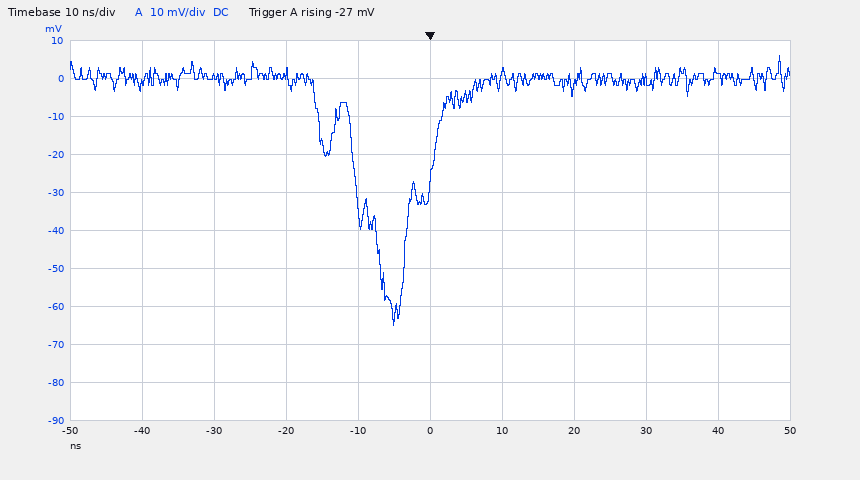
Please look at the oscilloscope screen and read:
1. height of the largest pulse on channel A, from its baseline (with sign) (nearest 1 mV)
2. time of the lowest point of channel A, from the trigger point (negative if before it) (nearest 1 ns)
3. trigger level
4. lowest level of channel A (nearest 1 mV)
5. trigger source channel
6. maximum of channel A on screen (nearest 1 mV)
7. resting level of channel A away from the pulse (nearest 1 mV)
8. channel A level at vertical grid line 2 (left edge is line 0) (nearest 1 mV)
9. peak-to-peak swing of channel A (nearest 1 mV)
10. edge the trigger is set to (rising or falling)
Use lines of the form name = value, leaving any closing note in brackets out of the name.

height of the largest pulse on channel A, from its baseline (with sign) = -65 mV
time of the lowest point of channel A, from the trigger point (negative if before it) = -5 ns
trigger level = -27 mV
lowest level of channel A = -65 mV
trigger source channel = channel A
maximum of channel A on screen = 6 mV
resting level of channel A away from the pulse = 0 mV
channel A level at vertical grid line 2 (left edge is line 0) = 1 mV
peak-to-peak swing of channel A = 71 mV
edge the trigger is set to = rising
